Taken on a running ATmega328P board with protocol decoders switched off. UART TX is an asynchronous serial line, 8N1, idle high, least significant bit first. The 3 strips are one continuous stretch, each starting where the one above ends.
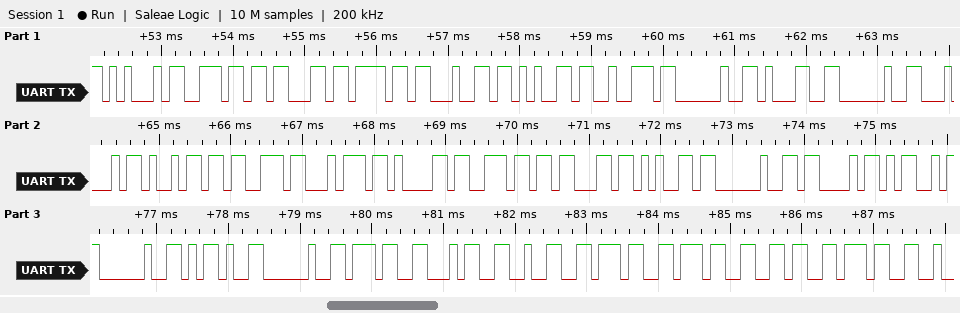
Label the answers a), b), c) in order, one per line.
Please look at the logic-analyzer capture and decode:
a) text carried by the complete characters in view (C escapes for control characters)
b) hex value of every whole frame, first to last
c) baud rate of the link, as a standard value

a) "Encoder 1 Distance CM - 7427767"
b) 45 6E 63 6F 64 65 72 20 31 20 44 69 73 74 61 6E 63 65 20 43 4D 20 2D 20 37 34 32 37 37 36 37
c) 9600 baud
